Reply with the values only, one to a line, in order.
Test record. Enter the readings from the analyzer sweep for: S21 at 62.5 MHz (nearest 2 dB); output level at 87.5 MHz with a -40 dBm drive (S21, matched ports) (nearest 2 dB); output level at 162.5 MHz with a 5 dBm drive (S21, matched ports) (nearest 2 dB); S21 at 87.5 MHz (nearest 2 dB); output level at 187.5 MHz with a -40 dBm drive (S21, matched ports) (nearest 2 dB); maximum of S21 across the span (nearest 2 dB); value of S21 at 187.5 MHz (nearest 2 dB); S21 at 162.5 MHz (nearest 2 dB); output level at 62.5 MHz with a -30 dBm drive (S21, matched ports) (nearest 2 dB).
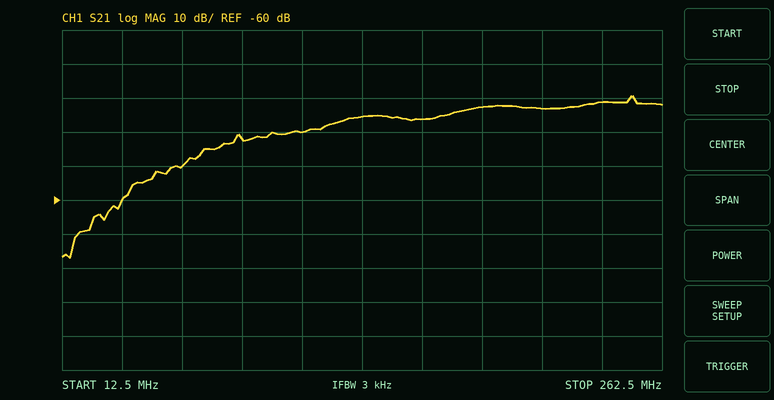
-50 dB
-82 dBm
-32 dBm
-42 dB
-72 dBm
-30 dB
-32 dB
-36 dB
-80 dBm
